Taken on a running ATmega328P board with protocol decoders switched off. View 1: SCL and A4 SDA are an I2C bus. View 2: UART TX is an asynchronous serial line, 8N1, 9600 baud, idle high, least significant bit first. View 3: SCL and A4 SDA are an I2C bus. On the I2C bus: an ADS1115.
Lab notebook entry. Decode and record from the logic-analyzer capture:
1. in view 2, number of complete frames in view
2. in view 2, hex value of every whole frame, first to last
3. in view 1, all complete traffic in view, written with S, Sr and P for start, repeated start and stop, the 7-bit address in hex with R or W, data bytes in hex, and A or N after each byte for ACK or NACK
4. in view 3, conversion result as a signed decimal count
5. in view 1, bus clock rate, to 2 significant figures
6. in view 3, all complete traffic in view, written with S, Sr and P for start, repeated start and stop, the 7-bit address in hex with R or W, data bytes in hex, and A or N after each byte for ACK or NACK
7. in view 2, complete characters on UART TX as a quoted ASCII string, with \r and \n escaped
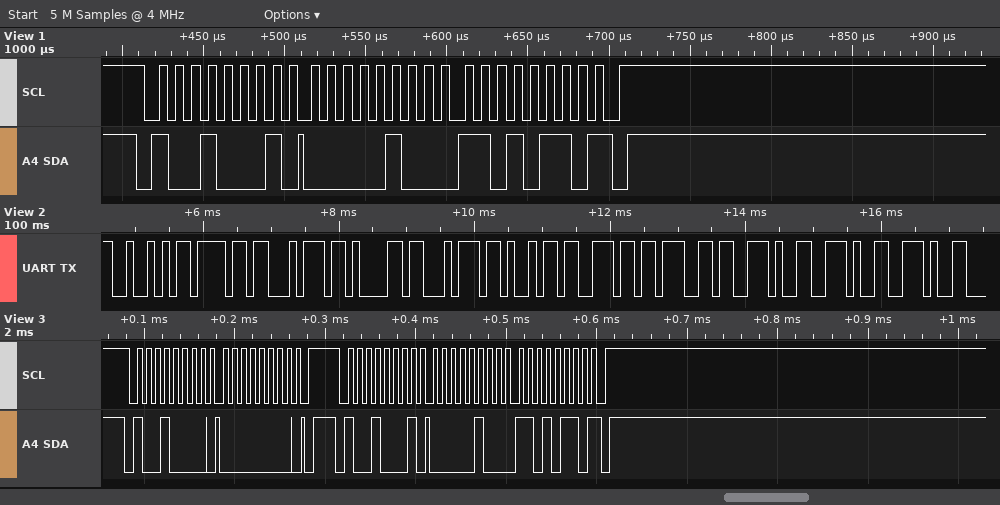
11
52 6F 74 61 74 69 6E 67 2E 2E 2E
S 48R A 04 A D6 N P
1238
100 kHz
S 48W A 00 A P S 48R A 04 A D6 N P
"Rotating..."
